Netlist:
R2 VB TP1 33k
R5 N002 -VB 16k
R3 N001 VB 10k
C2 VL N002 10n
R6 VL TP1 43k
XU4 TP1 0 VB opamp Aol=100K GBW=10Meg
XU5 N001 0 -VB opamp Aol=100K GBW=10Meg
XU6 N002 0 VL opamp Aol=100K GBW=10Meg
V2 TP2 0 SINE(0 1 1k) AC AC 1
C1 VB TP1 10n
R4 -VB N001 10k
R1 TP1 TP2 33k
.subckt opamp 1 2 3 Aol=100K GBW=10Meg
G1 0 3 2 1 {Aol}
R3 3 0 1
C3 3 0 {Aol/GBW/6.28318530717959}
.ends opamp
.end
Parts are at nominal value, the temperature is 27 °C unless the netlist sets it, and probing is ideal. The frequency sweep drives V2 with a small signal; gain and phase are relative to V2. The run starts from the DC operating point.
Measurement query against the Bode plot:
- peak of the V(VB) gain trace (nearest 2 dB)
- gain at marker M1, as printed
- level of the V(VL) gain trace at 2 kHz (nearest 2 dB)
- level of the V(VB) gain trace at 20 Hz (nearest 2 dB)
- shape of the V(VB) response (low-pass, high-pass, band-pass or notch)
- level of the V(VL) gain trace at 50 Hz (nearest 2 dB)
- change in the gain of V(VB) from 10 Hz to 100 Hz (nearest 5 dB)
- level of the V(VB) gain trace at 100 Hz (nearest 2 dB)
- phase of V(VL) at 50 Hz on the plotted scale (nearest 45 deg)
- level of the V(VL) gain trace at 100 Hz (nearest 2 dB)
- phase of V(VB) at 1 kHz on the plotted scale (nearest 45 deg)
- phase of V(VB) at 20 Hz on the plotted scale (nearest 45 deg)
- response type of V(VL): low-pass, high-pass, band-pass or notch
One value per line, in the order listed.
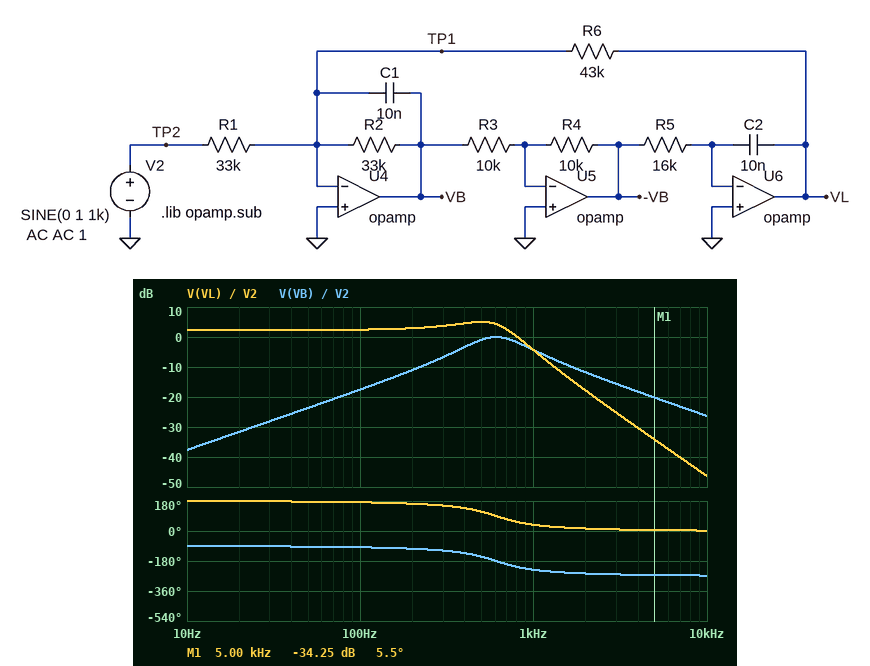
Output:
0 dB
-34.25 dB
-18 dB
-32 dB
band-pass
2 dB
20 dB
-18 dB
180 deg
2 dB
-225 deg
-90 deg
low-pass
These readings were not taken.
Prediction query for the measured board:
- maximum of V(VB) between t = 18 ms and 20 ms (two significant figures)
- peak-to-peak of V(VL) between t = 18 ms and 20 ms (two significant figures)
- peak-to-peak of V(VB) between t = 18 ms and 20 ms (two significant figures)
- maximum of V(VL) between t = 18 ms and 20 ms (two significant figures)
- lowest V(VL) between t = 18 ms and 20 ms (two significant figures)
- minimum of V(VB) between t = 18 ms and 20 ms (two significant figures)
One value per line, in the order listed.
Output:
610 mV
1.2 V
1.2 V
600 mV
-600 mV
-610 mV
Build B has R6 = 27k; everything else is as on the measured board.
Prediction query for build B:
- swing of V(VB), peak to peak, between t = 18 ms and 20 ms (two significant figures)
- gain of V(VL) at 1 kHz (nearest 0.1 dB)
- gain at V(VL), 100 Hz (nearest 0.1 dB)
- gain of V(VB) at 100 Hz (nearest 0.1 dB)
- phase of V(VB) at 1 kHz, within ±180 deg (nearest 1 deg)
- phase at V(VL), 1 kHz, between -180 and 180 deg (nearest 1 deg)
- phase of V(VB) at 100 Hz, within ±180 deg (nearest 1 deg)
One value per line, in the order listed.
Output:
1.5 V
-2.4 dB
-1.6 dB
-21.6 dB
139 deg
49 deg
-95 deg
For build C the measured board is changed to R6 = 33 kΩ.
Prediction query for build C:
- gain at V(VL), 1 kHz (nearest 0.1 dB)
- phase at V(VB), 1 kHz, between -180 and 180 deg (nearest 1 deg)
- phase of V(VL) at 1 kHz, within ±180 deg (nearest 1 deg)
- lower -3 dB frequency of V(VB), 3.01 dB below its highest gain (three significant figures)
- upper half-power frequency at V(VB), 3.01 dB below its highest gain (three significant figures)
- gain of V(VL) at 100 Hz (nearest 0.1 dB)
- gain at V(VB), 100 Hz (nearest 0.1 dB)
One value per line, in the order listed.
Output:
-3.4 dB
133 deg
43 deg
492 Hz
974 Hz
0.1 dB
-19.8 dB
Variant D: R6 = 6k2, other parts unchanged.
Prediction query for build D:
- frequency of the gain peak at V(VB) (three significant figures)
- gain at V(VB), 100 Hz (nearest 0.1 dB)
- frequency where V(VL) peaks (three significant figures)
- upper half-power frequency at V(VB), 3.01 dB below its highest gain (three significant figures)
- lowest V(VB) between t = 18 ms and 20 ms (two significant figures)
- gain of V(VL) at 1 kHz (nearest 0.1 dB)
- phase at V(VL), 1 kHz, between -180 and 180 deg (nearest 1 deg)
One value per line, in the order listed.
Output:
1.60 kHz
-34.4 dB
1.56 kHz
1.86 kHz
-300 mV
-10.6 dB
163 deg
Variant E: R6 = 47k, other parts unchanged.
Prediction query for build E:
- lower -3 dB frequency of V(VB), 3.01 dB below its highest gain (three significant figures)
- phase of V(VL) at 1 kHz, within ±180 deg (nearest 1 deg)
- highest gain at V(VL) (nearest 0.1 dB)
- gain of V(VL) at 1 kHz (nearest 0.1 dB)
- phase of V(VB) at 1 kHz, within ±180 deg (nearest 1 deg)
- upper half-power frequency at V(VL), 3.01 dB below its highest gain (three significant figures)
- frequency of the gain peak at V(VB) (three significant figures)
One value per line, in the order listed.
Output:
387 Hz
36 deg
5.5 dB
-4.7 dB
126 deg
689 Hz
580 Hz
